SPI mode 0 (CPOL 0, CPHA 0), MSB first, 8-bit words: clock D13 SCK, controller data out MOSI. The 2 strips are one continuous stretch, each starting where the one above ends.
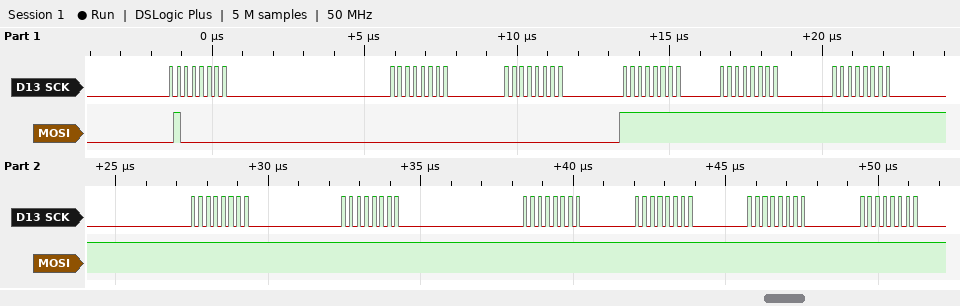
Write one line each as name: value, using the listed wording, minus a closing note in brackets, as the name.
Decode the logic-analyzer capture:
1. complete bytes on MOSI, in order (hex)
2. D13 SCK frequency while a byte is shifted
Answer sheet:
complete bytes on MOSI, in order: 40 00 00 FF FF FF FF FF FF FF FF FF
D13 SCK frequency while a byte is shifted: 4 MHz
